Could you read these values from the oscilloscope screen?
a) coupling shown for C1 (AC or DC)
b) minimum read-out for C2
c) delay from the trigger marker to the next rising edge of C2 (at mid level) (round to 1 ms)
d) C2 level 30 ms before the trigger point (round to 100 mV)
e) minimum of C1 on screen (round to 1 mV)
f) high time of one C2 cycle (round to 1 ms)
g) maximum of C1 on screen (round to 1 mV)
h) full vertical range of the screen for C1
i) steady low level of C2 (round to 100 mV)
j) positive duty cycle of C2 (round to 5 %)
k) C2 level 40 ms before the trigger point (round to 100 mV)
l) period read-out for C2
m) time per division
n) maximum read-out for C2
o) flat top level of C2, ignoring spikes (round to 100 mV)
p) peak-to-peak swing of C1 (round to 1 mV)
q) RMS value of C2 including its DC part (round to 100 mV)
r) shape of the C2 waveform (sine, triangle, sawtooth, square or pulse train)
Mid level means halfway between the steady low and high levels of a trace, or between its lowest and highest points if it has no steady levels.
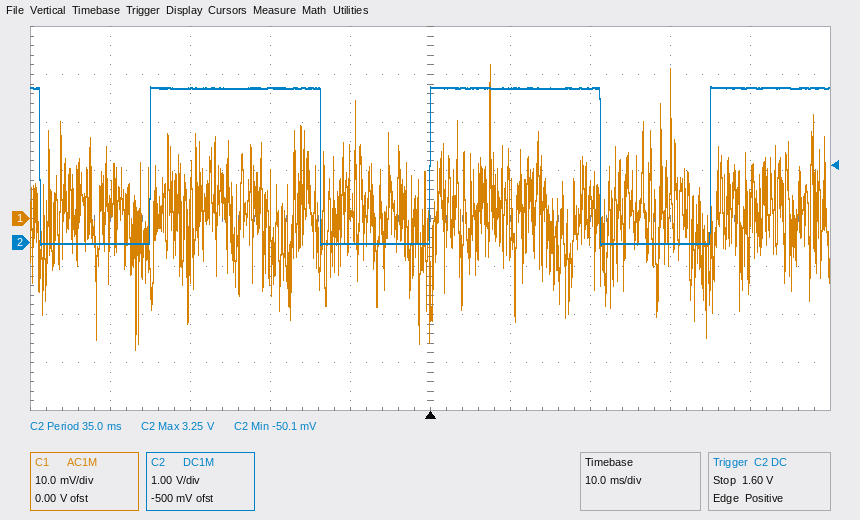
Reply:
AC
-50.1 mV
35 ms
3.2 V
-27 mV
21 ms
32 mV
80 mV
0.0 V
60 %
0.0 V
35.0 ms
10 ms
3.25 V
3.2 V
59 mV
2.5 V
pulse train
